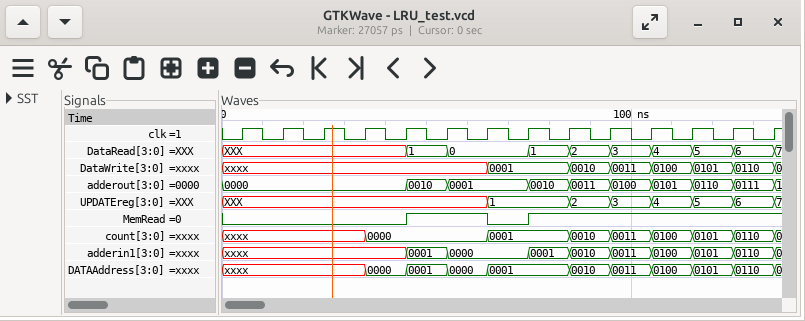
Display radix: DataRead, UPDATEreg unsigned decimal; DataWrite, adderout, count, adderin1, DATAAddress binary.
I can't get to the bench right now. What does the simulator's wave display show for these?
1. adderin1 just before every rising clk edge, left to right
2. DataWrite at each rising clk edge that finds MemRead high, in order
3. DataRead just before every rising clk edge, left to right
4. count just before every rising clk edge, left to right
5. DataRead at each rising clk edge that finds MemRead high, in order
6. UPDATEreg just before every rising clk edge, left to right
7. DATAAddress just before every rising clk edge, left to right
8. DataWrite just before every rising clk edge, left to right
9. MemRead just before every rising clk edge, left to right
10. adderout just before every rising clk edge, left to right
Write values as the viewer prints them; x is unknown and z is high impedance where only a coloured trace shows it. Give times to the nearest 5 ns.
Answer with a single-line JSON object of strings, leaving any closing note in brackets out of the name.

{"adderin1 just before every rising clk edge, left to right": "xxxx, xxxx, xxxx, xxxx, xxxx, 0001, 0000, 0000, 0001, 0010, 0011, 0100, 0101, 0110", "DataWrite at each rising clk edge that finds MemRead high, in order": "xxxx, xxxx, 0001, 0010, 0011, 0100, 0101, 0110", "DataRead just before every rising clk edge, left to right": "XXX, XXX, XXX, XXX, XXX, 1, 0, 0, 1, 2, 3, 4, 5, 6", "count just before every rising clk edge, left to right": "xxxx, xxxx, xxxx, xxxx, 0000, 0000, 0000, 0001, 0001, 0010, 0011, 0100, 0101, 0110", "DataRead at each rising clk edge that finds MemRead high, in order": "1, 0, 1, 2, 3, 4, 5, 6", "UPDATEreg just before every rising clk edge, left to right": "XXX, XXX, XXX, XXX, XXX, XXX, XXX, 1, 1, 2, 3, 4, 5, 6", "DATAAddress just before every rising clk edge, left to right": "xxxx, xxxx, xxxx, xxxx, 0000, 0001, 0000, 0001, 0001, 0010, 0011, 0100, 0101, 0110", "DataWrite just before every rising clk edge, left to right": "xxxx, xxxx, xxxx, xxxx, xxxx, xxxx, xxxx, 0001, 0001, 0010, 0011, 0100, 0101, 0110", "MemRead just before every rising clk edge, left to right": "0 0 0 0 0 1 1 0 1 1 1 1 1 1", "adderout just before every rising clk edge, left to right": "0000, 0000, 0000, 0000, 0000, 0010, 0001, 0001, 0010, 0011, 0100, 0101, 0110, 0111"}
